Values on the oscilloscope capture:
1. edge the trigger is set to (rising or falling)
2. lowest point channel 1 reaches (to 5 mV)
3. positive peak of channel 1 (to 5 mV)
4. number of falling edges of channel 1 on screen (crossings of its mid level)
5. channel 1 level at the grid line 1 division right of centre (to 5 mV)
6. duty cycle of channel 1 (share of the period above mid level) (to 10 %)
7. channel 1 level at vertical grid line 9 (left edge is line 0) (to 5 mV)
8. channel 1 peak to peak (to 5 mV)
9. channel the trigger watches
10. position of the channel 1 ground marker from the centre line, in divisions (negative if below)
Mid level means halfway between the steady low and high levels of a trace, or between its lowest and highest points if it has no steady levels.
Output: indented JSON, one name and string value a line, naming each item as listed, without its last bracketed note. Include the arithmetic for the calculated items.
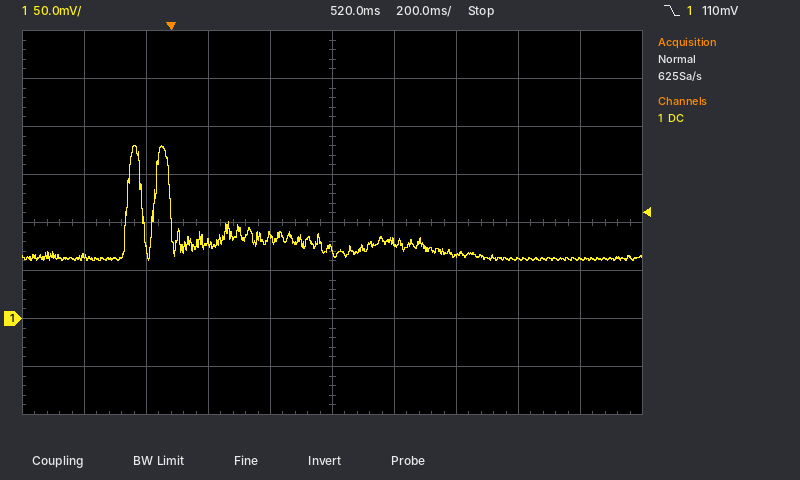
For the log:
{
  "edge the trigger is set to": "falling",
  "lowest point channel 1 reaches": "60 mV",
  "positive peak of channel 1": "180 mV",
  "number of falling edges of channel 1 on screen": "2",
  "channel 1 level at the grid line 1 division right of centre": "80 mV",
  "duty cycle of channel 1 (share of the period above mid level)": "60 %",
  "channel 1 level at vertical grid line 9 (left edge is line 0)": "60 mV",
  "channel 1 peak to peak": "180 mV − (60 mV) = 120 mV",
  "channel the trigger watches": "channel 1",
  "position of the channel 1 ground marker from the centre line, in divisions": "-2.0 div"
}
